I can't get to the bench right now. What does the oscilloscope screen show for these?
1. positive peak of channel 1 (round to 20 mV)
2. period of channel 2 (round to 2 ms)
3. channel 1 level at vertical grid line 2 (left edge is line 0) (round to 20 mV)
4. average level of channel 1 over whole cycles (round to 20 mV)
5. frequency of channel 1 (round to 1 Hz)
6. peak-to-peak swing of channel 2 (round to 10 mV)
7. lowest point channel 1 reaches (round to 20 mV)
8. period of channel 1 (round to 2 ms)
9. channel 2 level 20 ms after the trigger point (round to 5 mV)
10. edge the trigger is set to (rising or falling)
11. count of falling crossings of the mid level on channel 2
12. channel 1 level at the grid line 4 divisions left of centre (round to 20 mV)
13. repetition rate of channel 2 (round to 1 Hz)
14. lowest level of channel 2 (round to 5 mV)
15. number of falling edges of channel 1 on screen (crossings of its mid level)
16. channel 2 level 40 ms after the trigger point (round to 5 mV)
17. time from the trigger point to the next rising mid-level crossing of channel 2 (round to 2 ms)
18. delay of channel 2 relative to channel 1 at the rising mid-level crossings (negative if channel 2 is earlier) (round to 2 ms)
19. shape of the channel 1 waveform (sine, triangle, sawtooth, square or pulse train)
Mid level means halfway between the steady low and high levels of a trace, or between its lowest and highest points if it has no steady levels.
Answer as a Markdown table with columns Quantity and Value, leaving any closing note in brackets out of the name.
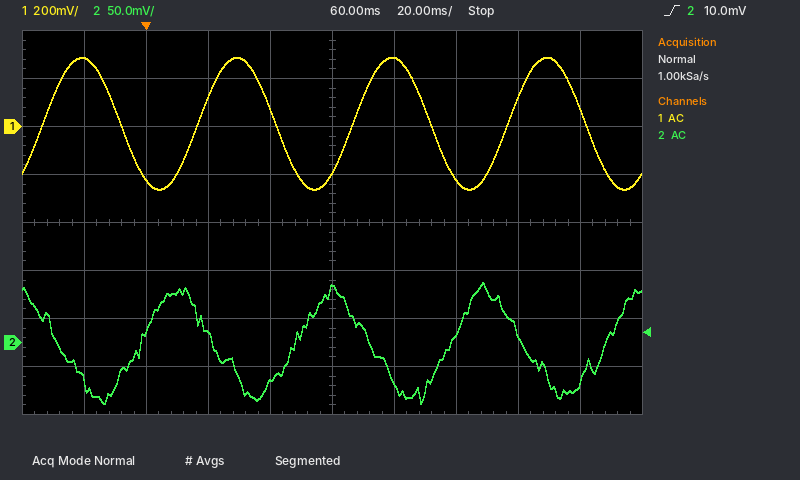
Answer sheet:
| Quantity | Value |
|---|---|
| positive peak of channel 1 | 280 mV |
| period of channel 2 | 50 ms |
| channel 1 level at vertical grid line 2 (left edge is line 0) | -220 mV |
| average level of channel 1 over whole cycles | 20 mV |
| frequency of channel 1 | 20 Hz |
| peak-to-peak swing of channel 2 | 130 mV |
| lowest point channel 1 reaches | -260 mV |
| period of channel 1 | 50 ms |
| channel 2 level 20 ms after the trigger point | 10 mV |
| edge the trigger is set to | rising |
| count of falling crossings of the mid level on channel 2 | 4 |
| channel 1 level at the grid line 4 divisions left of centre | 280 mV |
| repetition rate of channel 2 | 20 Hz |
| lowest level of channel 2 | -65 mV |
| number of falling edges of channel 1 on screen | 4 |
| channel 2 level 40 ms after the trigger point | -40 mV |
| time from the trigger point to the next rising mid-level crossing of channel 2 | 48 ms |
| delay of channel 2 relative to channel 1 at the rising mid-level crossings (negative if channel 2 is earlier) | -18 ms |
| shape of the channel 1 waveform | sine |
